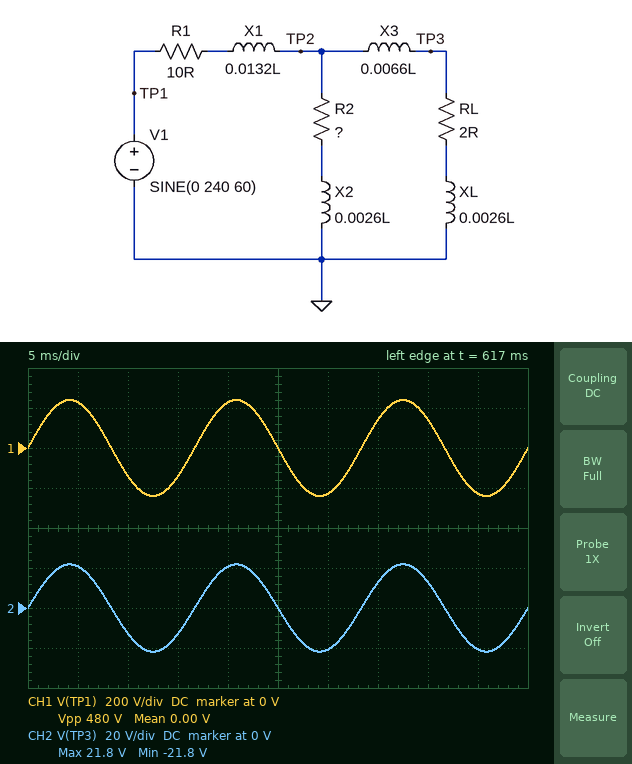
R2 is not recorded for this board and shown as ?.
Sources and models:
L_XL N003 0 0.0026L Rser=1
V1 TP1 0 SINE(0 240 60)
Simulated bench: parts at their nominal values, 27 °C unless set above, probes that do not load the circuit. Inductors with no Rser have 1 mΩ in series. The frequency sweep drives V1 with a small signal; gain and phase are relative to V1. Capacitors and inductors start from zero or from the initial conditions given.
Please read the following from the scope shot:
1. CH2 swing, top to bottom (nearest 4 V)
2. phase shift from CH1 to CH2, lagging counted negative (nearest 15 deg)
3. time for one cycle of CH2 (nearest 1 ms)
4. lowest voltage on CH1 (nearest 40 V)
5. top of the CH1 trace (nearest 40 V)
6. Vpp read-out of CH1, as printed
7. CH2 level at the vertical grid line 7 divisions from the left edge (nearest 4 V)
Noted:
44 V
0 deg
17 ms
-240 V
240 V
480 V
12 V
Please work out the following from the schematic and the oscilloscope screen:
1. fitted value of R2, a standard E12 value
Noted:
1.5 Ω
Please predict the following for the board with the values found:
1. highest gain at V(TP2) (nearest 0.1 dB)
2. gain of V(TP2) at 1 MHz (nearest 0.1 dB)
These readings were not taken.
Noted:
-17.5 dB
-17.5 dB
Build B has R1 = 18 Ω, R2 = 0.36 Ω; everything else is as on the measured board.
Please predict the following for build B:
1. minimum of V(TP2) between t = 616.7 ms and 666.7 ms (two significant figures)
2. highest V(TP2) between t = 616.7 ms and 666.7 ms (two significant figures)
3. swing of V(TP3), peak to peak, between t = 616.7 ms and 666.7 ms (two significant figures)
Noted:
-4.2 V
4.2 V
8.4 V
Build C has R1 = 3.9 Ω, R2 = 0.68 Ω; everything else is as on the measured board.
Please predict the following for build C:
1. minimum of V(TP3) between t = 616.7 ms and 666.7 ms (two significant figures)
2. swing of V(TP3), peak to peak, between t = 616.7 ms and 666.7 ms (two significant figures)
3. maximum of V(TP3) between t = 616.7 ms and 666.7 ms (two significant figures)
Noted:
-30 V
60 V
30 V
